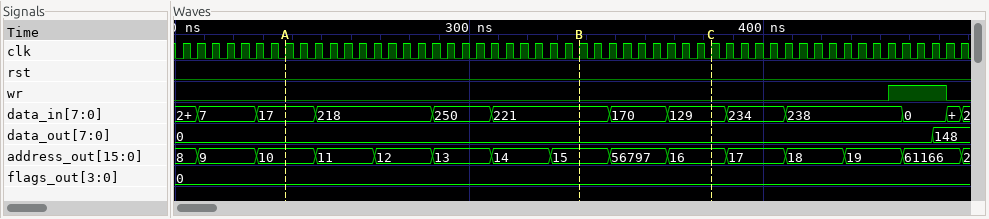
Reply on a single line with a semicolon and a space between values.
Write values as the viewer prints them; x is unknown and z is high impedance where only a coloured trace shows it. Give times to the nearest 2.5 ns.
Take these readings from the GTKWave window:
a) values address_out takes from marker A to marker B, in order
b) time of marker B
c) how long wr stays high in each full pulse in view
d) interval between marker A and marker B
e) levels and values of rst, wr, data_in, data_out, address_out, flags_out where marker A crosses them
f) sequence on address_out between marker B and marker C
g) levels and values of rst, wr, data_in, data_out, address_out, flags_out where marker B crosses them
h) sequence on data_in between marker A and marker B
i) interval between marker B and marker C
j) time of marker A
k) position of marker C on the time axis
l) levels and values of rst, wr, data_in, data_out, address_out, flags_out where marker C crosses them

10, 11, 12, 13, 14, 15; 337.5 ns; 20 ns; 100 ns; rst=0, wr=0, data_in=17, data_out=0, address_out=10, flags_out=0; 15, 56797, 16; rst=0, wr=0, data_in=221, data_out=0, address_out=15, flags_out=0; 17, 218, 250, 221; 45 ns; 237.5 ns; 382.5 ns; rst=0, wr=0, data_in=129, data_out=0, address_out=16, flags_out=0
